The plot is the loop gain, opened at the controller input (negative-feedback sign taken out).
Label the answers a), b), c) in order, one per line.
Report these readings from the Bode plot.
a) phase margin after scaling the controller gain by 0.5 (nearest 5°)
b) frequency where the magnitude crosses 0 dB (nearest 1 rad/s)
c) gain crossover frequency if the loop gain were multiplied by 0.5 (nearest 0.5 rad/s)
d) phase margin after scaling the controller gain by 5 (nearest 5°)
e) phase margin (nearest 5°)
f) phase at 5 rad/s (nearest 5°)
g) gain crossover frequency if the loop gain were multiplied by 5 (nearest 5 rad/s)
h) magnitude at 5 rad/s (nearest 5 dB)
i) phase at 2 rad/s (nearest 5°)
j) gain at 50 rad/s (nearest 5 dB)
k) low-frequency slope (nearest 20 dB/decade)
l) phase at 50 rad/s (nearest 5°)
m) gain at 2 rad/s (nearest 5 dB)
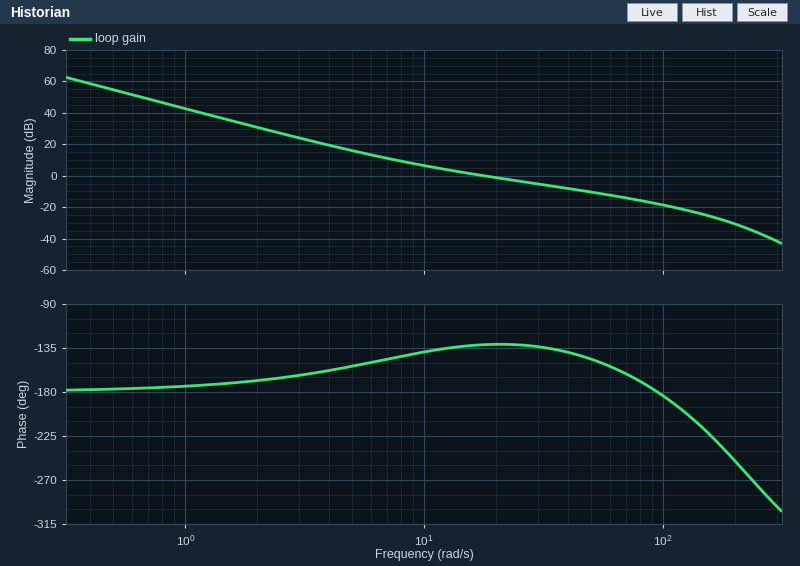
a) 40°
b) 18 rad/s
c) 10.5 rad/s
d) 20°
e) 50°
f) -155°
g) 70 rad/s
h) 15 dB
i) -170°
j) -10 dB
k) -40 dB/decade
l) -145°
m) 30 dB
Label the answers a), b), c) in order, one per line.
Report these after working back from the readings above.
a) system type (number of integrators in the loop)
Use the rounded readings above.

a) 2
